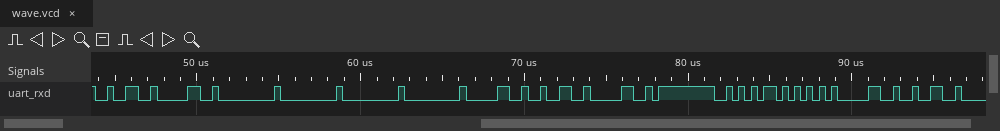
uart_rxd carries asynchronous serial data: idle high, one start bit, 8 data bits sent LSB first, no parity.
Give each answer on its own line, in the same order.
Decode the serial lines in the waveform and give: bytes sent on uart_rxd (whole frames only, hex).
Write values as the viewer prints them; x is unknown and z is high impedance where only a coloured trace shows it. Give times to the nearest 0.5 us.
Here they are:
32, 30, 00, 00, 00, 00, 30, 32, 30, FF, AA, 55, 30, 32
